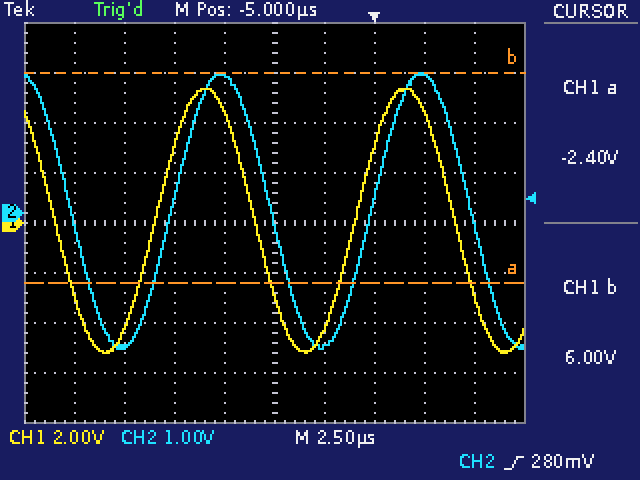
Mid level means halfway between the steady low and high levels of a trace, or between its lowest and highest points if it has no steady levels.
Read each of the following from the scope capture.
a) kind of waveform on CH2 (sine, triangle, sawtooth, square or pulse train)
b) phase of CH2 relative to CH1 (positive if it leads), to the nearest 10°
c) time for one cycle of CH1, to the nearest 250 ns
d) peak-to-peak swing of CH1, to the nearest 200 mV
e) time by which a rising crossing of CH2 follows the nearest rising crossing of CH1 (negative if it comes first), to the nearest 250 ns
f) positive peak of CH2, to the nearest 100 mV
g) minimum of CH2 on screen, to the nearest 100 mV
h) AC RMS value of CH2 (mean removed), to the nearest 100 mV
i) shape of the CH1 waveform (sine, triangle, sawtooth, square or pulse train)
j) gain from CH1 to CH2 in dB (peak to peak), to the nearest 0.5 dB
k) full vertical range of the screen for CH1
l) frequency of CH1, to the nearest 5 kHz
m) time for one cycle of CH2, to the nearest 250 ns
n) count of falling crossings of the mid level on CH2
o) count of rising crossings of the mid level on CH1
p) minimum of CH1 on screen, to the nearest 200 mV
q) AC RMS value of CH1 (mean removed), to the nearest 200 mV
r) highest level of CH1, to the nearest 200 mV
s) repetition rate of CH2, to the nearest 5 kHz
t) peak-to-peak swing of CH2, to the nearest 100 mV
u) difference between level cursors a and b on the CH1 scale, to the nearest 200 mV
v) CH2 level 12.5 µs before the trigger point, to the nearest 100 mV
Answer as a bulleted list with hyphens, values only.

- sine
- -30°
- 10.00 µs
- 10.6 V
- +750 ns
- 2.8 V
- -2.7 V
- 1.9 V
- sine
- -5.5 dB
- 16 V
- 100 kHz
- 10.00 µs
- 3
- 2
- -5.2 V
- 3.8 V
- 5.4 V
- 100 kHz
- 5.5 V
- 8.4 V
- -2.7 V
